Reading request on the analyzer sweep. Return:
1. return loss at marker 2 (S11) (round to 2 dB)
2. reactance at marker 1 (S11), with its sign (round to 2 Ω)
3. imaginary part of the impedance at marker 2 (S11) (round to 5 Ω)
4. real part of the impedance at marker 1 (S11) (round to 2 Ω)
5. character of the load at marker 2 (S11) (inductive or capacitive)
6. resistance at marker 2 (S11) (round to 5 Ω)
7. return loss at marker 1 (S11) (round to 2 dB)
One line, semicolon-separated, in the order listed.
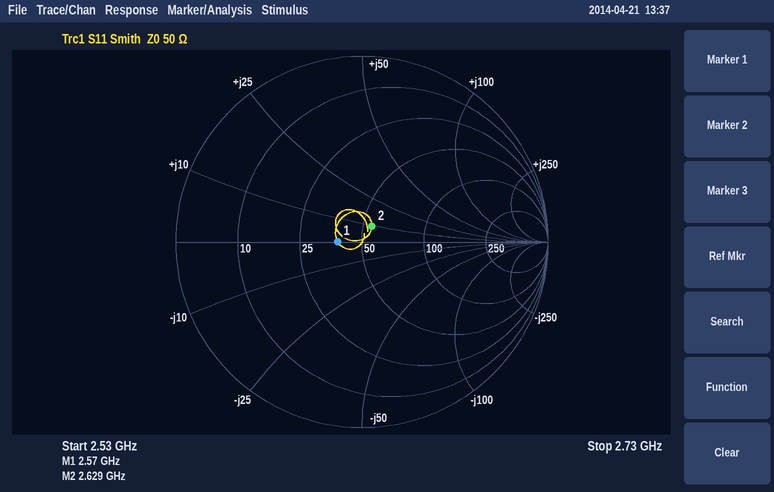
20 dB; 0 Ω; +10 Ω; 38 Ω; inductive; 55 Ω; 18 dB
